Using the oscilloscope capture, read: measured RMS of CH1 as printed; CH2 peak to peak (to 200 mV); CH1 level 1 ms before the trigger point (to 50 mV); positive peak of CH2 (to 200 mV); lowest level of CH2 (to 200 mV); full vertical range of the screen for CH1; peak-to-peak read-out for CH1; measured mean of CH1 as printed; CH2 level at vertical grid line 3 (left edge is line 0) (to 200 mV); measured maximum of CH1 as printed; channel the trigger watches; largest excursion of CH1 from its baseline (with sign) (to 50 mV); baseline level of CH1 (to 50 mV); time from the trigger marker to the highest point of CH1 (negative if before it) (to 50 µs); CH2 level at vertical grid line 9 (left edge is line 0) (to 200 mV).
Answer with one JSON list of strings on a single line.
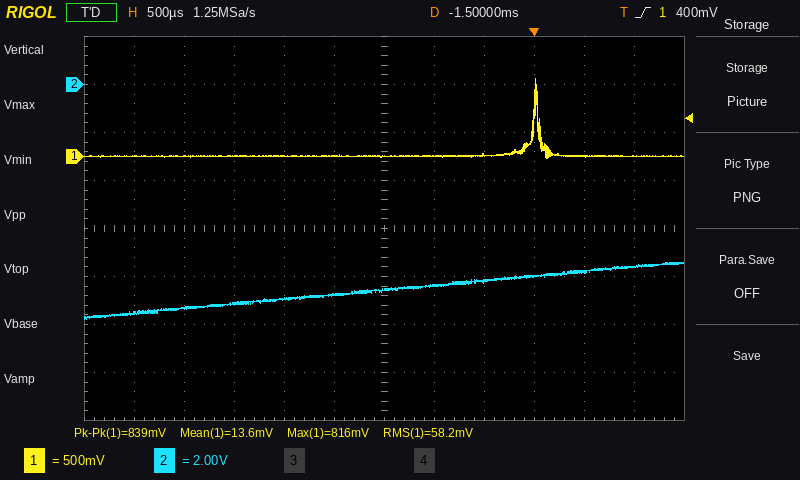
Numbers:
["58.2 mV", "2.4 V", "0 mV", "-7.4 V", "-9.8 V", "4 V", "839 mV", "13.6 mV", "-9.2 V", "816 mV", "CH1", "+800 mV", "0 mV", "0 µs", "-8.0 V"]
